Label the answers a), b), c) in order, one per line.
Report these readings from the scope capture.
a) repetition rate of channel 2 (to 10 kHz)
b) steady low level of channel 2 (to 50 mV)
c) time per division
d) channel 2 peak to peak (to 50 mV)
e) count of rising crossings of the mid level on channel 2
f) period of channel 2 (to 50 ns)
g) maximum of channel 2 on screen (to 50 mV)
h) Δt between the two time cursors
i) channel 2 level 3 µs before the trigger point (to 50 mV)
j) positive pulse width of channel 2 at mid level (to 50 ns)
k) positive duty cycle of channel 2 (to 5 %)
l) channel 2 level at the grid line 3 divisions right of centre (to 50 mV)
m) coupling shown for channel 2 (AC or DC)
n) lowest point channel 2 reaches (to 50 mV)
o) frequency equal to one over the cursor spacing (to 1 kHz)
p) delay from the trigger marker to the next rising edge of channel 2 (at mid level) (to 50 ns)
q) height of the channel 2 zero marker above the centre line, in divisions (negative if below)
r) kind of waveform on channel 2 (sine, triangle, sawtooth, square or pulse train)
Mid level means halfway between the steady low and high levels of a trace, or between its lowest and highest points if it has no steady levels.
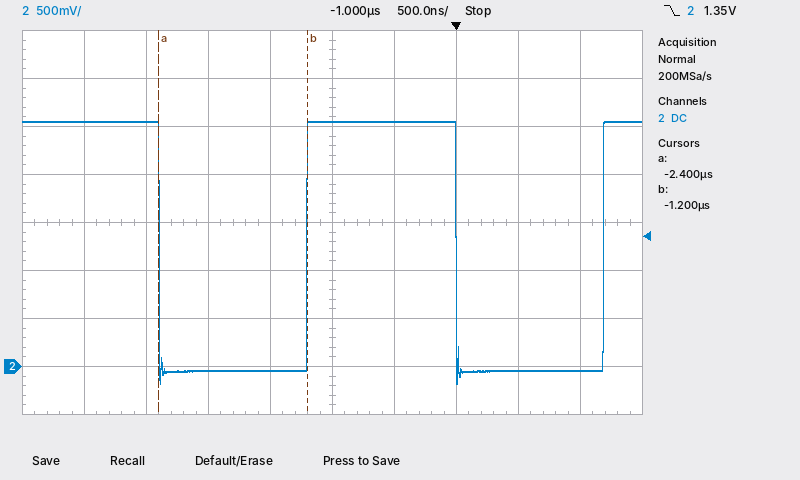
a) 420 kHz
b) -50 mV
c) 500 ns
d) 2.75 V
e) 2
f) 2.40 µs
g) 2.55 V
h) 1.20 µs
i) 2.55 V
j) 1.20 µs
k) 50 %
l) -50 mV
m) DC
n) -200 mV
o) 833 kHz
p) 1.20 µs
q) -3.0 div
r) square
